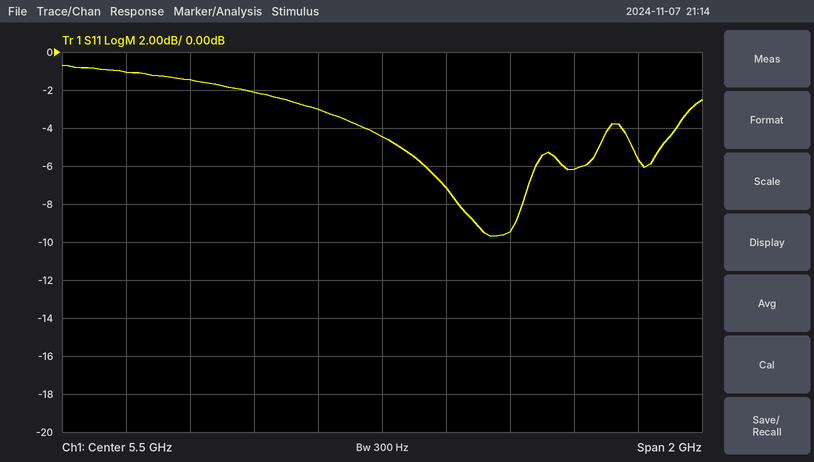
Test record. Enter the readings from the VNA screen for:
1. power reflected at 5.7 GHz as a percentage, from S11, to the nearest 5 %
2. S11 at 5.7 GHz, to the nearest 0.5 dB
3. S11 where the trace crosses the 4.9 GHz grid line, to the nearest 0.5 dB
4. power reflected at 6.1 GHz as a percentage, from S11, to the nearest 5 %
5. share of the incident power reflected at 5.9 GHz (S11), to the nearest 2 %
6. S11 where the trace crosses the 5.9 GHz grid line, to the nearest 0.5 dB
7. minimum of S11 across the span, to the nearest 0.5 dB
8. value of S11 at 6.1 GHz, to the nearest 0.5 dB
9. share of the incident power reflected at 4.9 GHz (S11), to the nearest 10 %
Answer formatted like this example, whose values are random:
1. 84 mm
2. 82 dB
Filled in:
1. 20 %
2. -7.0 dB
3. -1.5 dB
4. 25 %
5. 12 %
6. -9.5 dB
7. -9.5 dB
8. -6.0 dB
9. 70 %
